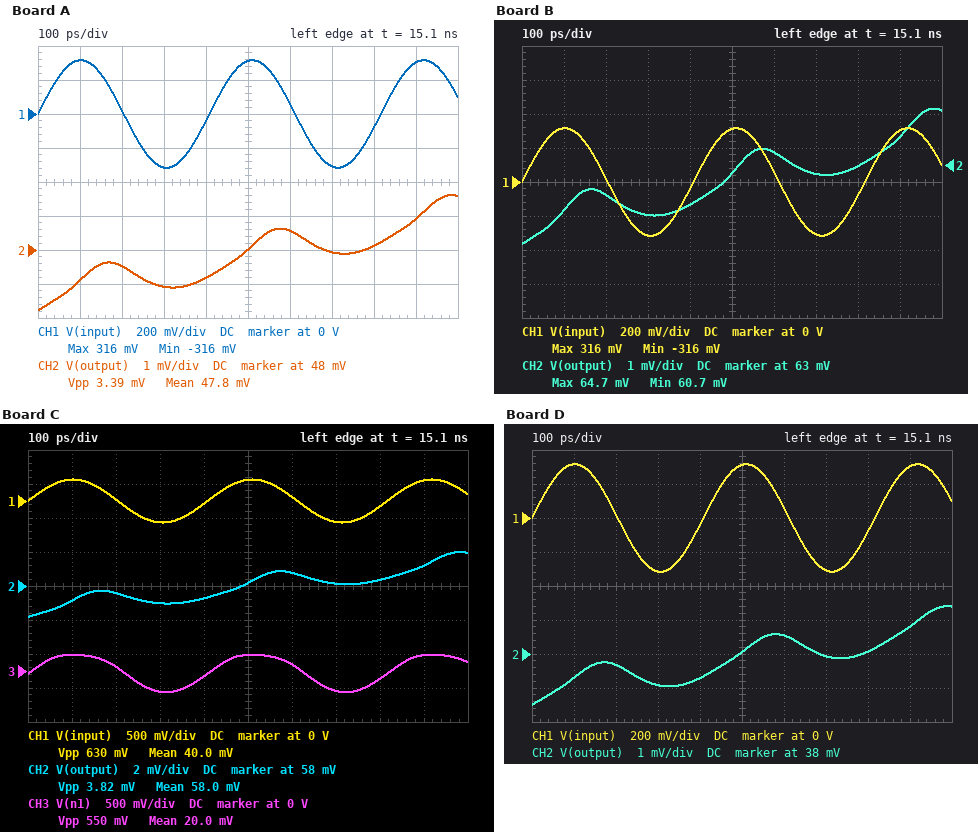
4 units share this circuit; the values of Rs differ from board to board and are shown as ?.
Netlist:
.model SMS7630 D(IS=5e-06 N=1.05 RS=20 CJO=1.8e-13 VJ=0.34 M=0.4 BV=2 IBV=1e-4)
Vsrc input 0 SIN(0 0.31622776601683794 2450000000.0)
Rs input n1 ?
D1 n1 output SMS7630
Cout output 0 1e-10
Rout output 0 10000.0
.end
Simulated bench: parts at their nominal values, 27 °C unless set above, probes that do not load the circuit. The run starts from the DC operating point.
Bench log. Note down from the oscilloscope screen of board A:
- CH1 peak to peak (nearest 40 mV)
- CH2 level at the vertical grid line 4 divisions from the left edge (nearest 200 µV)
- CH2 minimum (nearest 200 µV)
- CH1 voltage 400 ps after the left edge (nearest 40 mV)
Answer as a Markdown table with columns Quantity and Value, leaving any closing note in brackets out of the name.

| Quantity | Value |
|---|---|
| CH1 peak to peak | 640 mV |
| CH2 level at the vertical grid line 4 divisions from the left edge | 47.2 mV |
| CH2 minimum | 46.2 mV |
| CH1 voltage 400 ps after the left edge | -40 mV |
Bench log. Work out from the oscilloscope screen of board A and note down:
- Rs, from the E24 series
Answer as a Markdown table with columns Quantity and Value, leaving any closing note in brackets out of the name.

| Quantity | Value |
|---|---|
| Rs, from the E24 series | 82 Ω |
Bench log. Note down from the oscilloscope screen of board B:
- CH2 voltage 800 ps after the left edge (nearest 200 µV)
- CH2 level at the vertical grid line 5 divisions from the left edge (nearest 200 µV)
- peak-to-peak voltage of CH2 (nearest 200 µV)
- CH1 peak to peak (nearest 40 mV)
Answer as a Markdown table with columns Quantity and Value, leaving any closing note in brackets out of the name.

| Quantity | Value |
|---|---|
| CH2 voltage 800 ps after the left edge | 63.0 mV |
| CH2 level at the vertical grid line 5 divisions from the left edge | 62.8 mV |
| peak-to-peak voltage of CH2 | 4.0 mV |
| CH1 peak to peak | 640 mV |
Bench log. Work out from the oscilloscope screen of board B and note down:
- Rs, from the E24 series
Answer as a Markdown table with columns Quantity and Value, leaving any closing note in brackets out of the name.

| Quantity | Value |
|---|---|
| Rs, from the E24 series | 47 Ω |
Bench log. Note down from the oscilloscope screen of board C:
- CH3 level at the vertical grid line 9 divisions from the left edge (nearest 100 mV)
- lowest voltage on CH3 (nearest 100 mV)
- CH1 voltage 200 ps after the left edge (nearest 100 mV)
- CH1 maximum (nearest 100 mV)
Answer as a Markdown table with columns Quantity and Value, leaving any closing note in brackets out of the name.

| Quantity | Value |
|---|---|
| CH3 level at the vertical grid line 9 divisions from the left edge | 200 mV |
| lowest voltage on CH3 | -300 mV |
| CH1 voltage 200 ps after the left edge | 0 V |
| CH1 maximum | 300 mV |
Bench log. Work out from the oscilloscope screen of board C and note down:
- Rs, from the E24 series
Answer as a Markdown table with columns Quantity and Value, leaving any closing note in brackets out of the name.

| Quantity | Value |
|---|---|
| Rs, from the E24 series | 56 Ω |
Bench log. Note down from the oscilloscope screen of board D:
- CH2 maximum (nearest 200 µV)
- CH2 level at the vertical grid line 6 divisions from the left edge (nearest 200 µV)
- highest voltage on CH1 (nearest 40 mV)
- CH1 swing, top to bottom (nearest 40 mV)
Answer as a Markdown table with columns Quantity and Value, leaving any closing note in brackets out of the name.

| Quantity | Value |
|---|---|
| CH2 maximum | 39.4 mV |
| CH2 level at the vertical grid line 6 divisions from the left edge | 38.6 mV |
| highest voltage on CH1 | 320 mV |
| CH1 swing, top to bottom | 640 mV |
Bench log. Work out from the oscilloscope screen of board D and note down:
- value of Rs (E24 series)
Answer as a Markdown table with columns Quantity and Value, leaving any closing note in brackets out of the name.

| Quantity | Value |
|---|---|
| value of Rs | 120 Ω |
